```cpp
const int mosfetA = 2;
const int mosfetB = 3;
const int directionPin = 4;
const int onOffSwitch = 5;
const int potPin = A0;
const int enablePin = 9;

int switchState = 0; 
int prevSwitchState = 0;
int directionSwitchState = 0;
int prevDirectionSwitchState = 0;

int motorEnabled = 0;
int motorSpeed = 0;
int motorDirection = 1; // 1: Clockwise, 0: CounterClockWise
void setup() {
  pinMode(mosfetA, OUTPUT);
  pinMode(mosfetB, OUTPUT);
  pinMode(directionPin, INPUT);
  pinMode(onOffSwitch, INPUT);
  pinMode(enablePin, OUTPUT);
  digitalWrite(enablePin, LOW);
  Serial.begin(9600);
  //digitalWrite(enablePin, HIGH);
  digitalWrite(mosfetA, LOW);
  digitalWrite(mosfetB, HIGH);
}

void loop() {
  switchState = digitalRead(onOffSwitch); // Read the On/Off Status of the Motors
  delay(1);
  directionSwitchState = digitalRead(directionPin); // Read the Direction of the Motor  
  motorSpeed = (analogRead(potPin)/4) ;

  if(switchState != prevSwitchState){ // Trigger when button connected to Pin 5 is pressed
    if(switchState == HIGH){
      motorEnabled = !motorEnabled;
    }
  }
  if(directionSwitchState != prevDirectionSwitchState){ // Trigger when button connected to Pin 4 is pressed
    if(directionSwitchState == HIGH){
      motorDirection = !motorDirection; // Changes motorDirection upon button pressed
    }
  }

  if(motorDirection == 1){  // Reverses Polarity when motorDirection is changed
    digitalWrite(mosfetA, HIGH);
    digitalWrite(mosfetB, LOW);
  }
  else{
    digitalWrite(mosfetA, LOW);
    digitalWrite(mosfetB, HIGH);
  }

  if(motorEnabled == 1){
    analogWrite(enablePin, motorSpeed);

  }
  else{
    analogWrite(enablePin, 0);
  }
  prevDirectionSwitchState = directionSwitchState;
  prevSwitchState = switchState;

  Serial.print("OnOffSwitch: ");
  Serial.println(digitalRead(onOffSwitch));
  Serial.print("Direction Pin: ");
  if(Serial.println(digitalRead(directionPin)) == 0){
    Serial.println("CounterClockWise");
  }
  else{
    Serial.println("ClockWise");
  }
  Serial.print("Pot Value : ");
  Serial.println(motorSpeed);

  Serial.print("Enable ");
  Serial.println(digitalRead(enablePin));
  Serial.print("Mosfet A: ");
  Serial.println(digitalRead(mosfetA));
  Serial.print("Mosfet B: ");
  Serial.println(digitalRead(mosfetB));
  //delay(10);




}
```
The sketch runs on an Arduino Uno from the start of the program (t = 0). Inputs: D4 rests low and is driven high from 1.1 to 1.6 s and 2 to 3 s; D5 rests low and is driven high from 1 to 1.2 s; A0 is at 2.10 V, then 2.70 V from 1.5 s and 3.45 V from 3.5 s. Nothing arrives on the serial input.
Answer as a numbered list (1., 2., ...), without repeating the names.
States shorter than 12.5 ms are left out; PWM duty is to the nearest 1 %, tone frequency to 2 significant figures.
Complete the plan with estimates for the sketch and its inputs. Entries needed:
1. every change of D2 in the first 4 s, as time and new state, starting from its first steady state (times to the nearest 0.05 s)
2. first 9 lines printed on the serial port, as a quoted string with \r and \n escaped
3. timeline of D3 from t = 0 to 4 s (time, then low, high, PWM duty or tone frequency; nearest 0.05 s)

1. 0 s high; 1.15 s low; 2.05 s high
2. "OnOffSwitch: 0\r\nDirection Pin: 0\r\nClockWise\r\nPot Value : 107\r\nEnable 0\r\nMosfet A: 1\r\nMosfet B: 0\r\nOnOffSwitch: 0\r\nDirection Pin: 0\r\n"
3. 0 s low; 1.15 s high; 2.05 s low
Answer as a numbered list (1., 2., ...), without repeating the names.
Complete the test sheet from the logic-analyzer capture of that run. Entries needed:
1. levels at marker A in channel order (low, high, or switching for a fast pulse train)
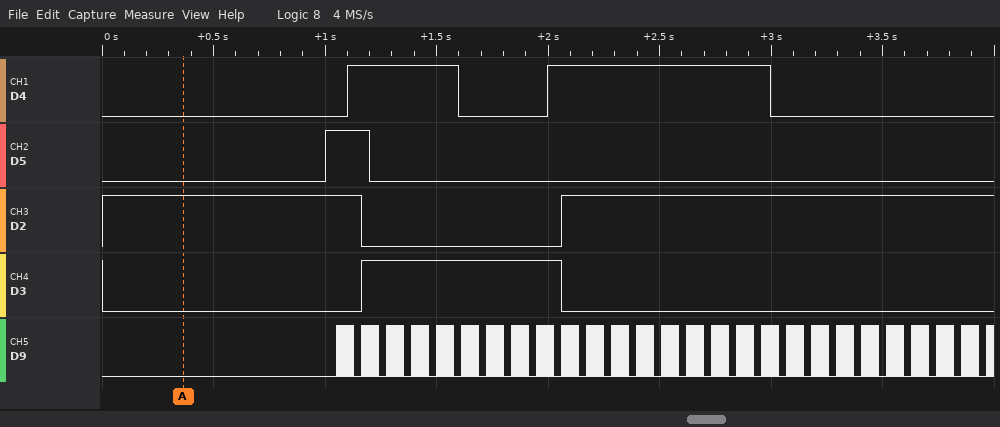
1. D4 low, D5 low, D2 high, D3 low, D9 low
